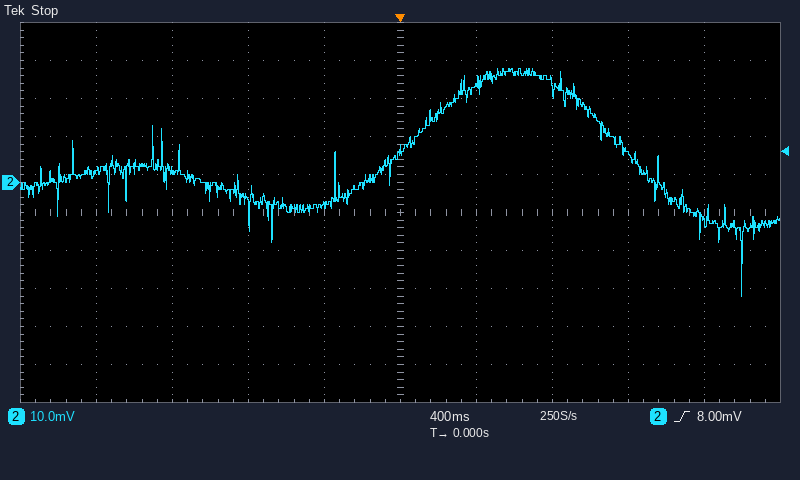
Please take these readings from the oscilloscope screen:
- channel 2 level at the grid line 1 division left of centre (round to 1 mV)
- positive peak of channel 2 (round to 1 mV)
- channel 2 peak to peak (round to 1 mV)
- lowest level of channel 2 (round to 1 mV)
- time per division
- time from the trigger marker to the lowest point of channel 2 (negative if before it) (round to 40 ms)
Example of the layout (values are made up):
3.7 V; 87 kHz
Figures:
-6 mV; 30 mV; 60 mV; -30 mV; 400 ms; +1.80 s
